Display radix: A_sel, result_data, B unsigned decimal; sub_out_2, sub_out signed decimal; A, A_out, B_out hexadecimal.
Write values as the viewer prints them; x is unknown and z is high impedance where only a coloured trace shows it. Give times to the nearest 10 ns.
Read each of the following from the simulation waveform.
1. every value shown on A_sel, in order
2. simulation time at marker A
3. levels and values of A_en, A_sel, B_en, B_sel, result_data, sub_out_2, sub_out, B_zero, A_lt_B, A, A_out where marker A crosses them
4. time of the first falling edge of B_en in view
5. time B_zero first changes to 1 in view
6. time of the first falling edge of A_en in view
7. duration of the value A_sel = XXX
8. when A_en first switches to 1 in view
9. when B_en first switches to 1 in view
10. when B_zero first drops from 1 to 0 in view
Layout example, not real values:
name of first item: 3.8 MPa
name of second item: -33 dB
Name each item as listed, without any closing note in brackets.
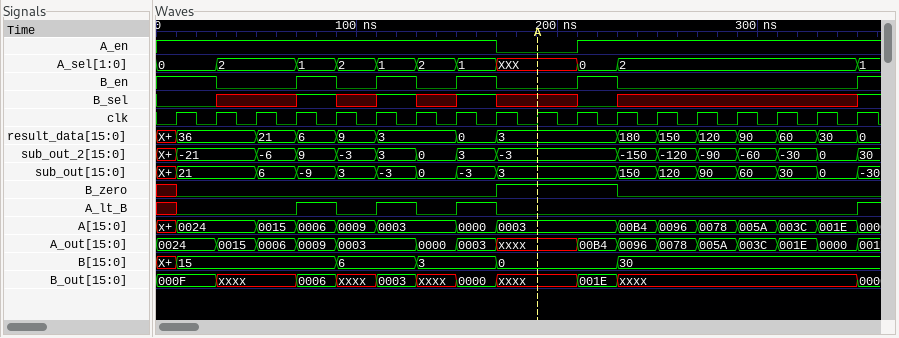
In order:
every value shown on A_sel, in order: 0, 2, 1, 2, 1, 2, 1, XXX, 0, 2, 1
simulation time at marker A: 190 ns
levels and values of A_en, A_sel, B_en, B_sel, result_data, sub_out_2, sub_out, B_zero, A_lt_B, A, A_out where marker A crosses them: A_en=0, A_sel=XXX, B_en=0, B_sel=x, result_data=3, sub_out_2=-3, sub_out=3, B_zero=1, A_lt_B=0, A=0003, A_out=xxxx
time of the first falling edge of B_en in view: 30 ns
time B_zero first changes to 1 in view: 170 ns
time of the first falling edge of A_en in view: 170 ns
duration of the value A_sel = XXX: 40 ns
when A_en first switches to 1 in view: 210 ns
when B_en first switches to 1 in view: 70 ns
when B_zero first drops from 1 to 0 in view: 230 ns
